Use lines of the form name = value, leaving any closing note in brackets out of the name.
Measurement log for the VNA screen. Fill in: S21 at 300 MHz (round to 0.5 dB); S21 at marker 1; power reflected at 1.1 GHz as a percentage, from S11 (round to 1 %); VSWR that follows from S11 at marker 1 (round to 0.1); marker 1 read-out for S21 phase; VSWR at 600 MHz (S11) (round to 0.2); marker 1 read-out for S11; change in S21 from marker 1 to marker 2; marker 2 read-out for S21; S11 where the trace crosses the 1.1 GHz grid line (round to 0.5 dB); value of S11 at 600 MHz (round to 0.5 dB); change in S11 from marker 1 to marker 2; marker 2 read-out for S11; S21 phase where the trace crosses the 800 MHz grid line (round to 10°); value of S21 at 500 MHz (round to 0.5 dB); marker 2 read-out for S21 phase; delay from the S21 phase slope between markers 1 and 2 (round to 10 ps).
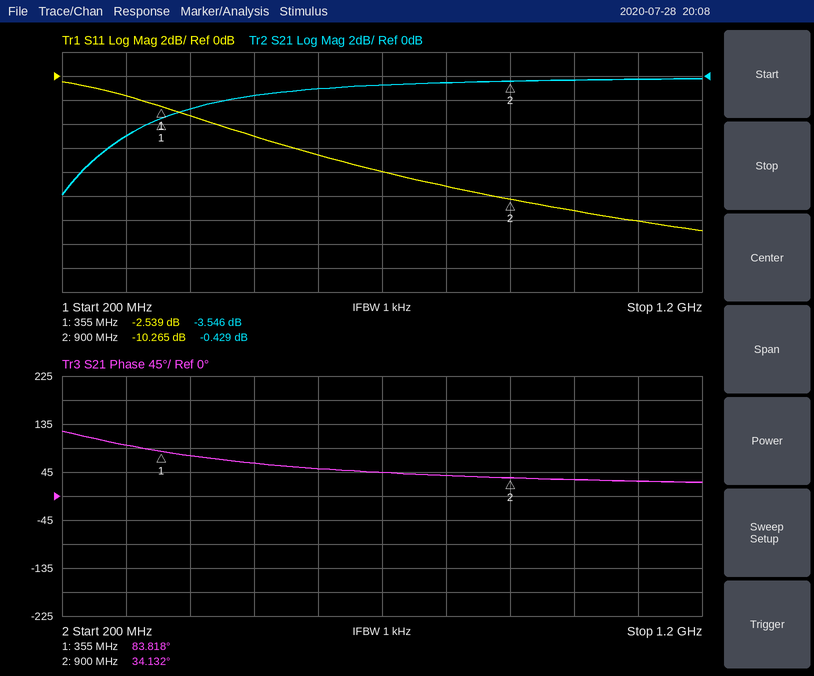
S21 at 300 MHz = -5.0 dB
S21 at marker 1 = -3.546 dB
power reflected at 1.1 GHz as a percentage, from S11 = 6 %
VSWR that follows from S11 at marker 1 = 6.9
marker 1 read-out for S21 phase = 83.818°
VSWR at 600 MHz (S11) = 2.8
marker 1 read-out for S11 = -2.539 dB
change in S21 from marker 1 to marker 2 = 3.117 dB
marker 2 read-out for S21 = -0.429 dB
S11 where the trace crosses the 1.1 GHz grid line = -12.0 dB
value of S11 at 600 MHz = -6.5 dB
change in S11 from marker 1 to marker 2 = -7.726 dB
marker 2 read-out for S11 = -10.265 dB
S21 phase where the trace crosses the 800 MHz grid line = 40°
value of S21 at 500 MHz = -1.5 dB
marker 2 read-out for S21 phase = 34.132°
delay from the S21 phase slope between markers 1 and 2 = 250 ps
